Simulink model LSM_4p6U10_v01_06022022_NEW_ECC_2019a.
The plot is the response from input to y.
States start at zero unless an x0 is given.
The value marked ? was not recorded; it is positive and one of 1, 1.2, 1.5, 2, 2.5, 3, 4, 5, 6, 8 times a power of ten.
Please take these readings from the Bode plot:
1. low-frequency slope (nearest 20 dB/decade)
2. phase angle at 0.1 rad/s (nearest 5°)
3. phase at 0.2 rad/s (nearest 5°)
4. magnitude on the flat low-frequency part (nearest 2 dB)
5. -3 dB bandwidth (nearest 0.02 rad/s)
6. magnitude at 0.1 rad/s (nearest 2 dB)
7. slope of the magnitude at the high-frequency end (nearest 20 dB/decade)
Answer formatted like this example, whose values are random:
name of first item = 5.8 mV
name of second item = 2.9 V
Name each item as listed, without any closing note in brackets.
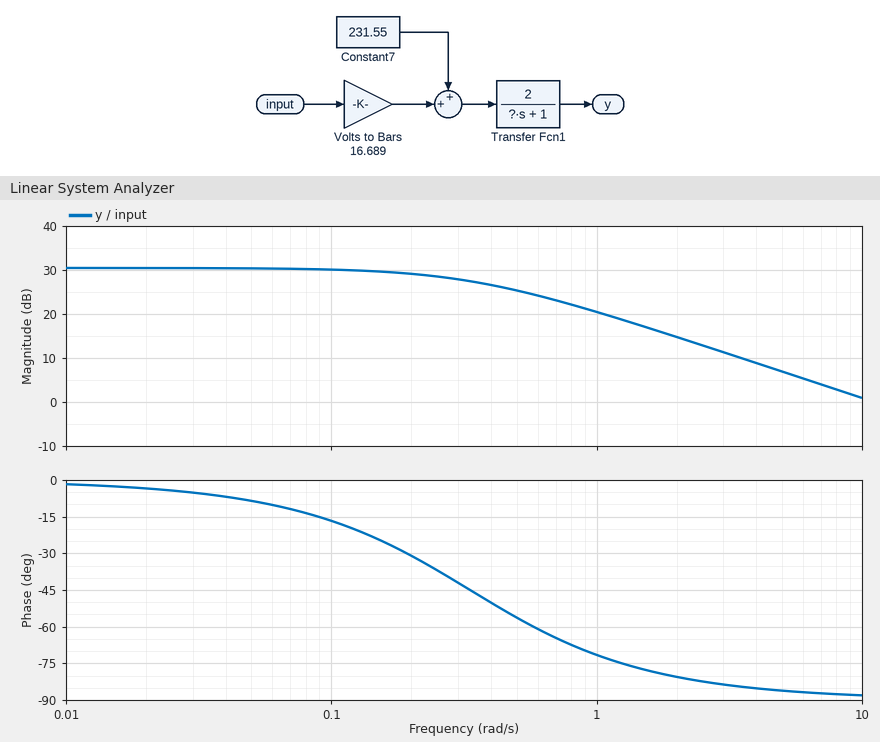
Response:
low-frequency slope = 0 dB/decade
phase angle at 0.1 rad/s = -15°
phase at 0.2 rad/s = -30°
magnitude on the flat low-frequency part = 30 dB
-3 dB bandwidth = 0.34 rad/s
magnitude at 0.1 rad/s = 30 dB
slope of the magnitude at the high-frequency end = -20 dB/decade
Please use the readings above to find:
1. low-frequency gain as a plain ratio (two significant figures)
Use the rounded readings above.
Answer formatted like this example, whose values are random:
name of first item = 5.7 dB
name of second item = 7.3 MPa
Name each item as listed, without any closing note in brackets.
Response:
low-frequency gain as a plain ratio = 32
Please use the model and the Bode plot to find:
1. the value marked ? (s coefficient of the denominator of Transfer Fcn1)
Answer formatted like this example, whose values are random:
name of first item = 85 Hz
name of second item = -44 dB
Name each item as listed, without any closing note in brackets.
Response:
the value marked ? = 3
